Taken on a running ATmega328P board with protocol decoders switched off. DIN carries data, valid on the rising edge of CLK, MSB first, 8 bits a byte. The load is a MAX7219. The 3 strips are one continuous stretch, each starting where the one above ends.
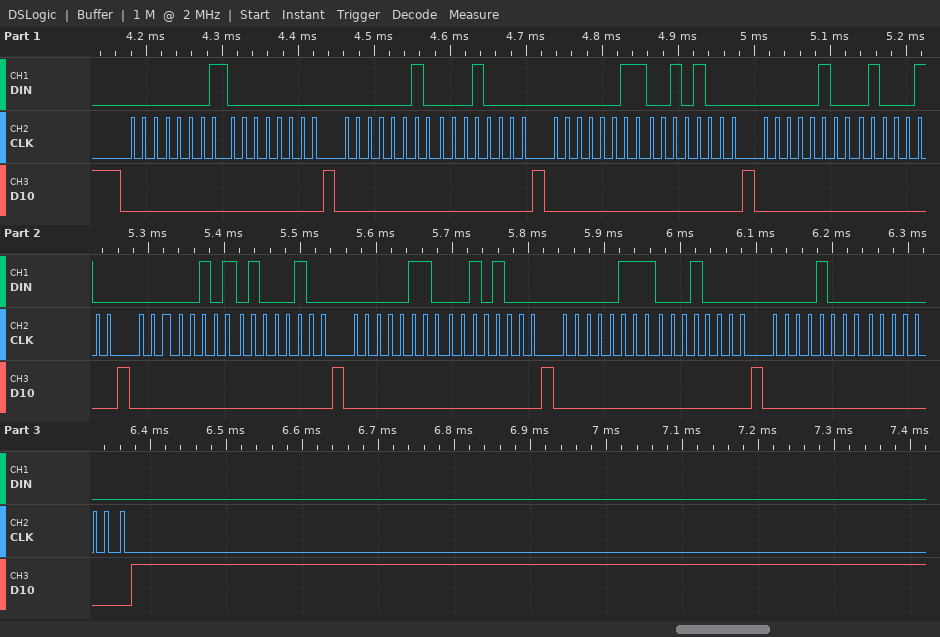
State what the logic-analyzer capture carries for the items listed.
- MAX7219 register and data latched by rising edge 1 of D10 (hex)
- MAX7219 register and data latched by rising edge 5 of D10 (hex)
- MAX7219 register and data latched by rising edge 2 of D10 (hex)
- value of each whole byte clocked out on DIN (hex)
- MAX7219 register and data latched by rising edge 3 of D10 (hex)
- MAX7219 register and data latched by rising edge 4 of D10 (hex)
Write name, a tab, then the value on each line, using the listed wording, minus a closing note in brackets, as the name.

MAX7219 register and data latched by rising edge 1 of D10	register 0x1, data 0x00
MAX7219 register and data latched by rising edge 5 of D10	register 0x5, data 0x44
MAX7219 register and data latched by rising edge 2 of D10	register 0x2, data 0x10
value of each whole byte clocked out on DIN	01 00 02 10 03 28 04 44 05 44 06 28 07 10 08 00
MAX7219 register and data latched by rising edge 3 of D10	register 0x3, data 0x28
MAX7219 register and data latched by rising edge 4 of D10	register 0x4, data 0x44
